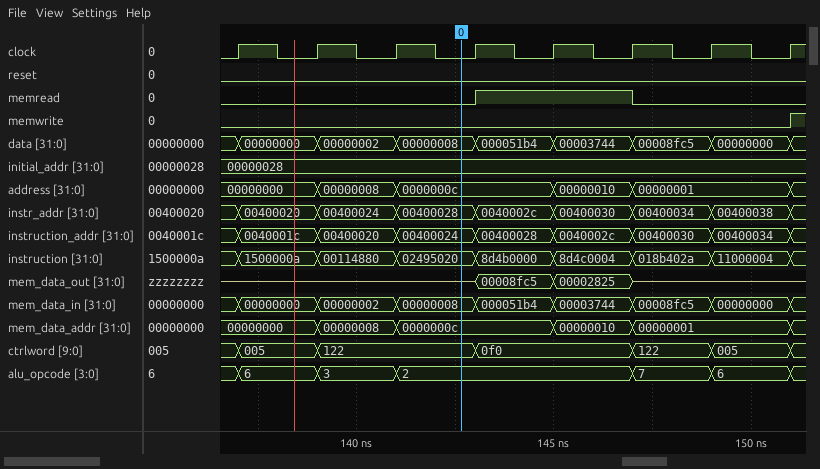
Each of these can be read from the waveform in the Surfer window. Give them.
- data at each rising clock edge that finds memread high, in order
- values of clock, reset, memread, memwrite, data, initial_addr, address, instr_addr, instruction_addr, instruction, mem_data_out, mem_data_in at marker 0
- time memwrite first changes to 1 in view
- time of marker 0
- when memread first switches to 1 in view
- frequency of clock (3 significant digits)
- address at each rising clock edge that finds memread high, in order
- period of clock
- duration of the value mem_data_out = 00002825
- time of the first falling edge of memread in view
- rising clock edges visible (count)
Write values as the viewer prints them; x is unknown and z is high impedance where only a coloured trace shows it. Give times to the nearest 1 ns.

000051b4, 00003744
clock=0, reset=0, memread=0, memwrite=0, data=00000008, initial_addr=00000028, address=0000000c, instr_addr=00400028, instruction_addr=00400024, instruction=02495020, mem_data_out=z, mem_data_in=00000008
151 ns
143 ns
143 ns
500 MHz
0000000c, 00000010
2 ns
2 ns
147 ns
8
